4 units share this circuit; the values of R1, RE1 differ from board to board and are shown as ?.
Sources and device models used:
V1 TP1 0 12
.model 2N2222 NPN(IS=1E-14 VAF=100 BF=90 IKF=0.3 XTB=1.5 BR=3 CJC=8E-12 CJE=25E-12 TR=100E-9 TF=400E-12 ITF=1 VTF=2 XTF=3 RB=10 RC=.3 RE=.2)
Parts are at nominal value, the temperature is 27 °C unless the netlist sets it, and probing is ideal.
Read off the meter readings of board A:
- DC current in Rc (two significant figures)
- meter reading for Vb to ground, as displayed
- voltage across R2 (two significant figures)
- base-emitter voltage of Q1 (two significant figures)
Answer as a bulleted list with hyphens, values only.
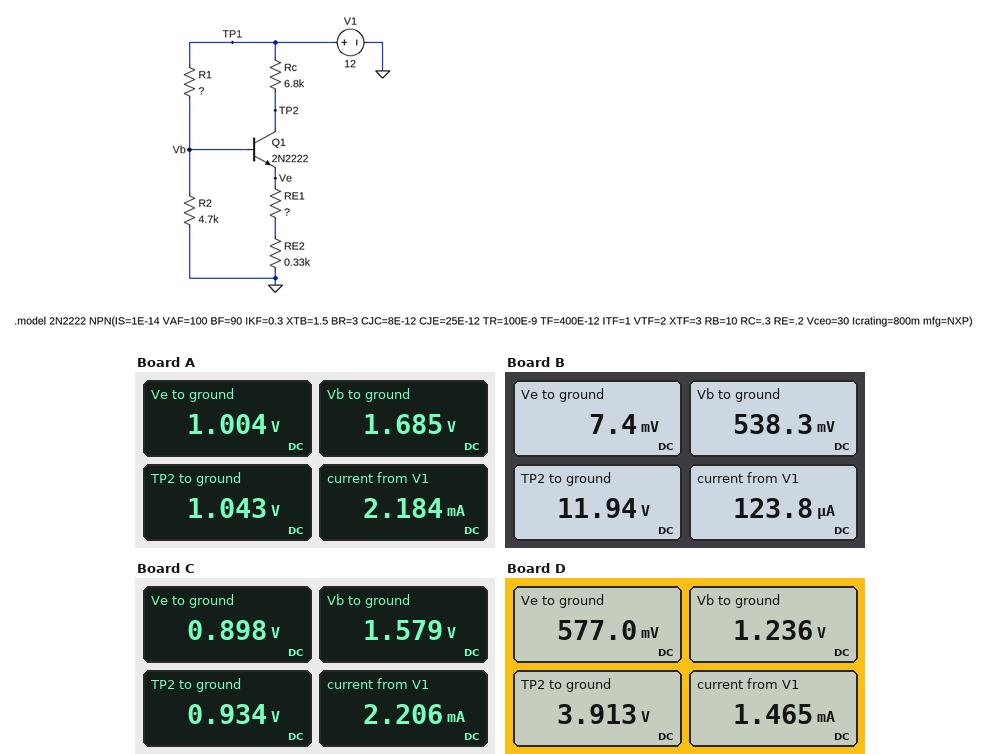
- 1.6 mA
- 1.685 V
- 1.7 V
- 680 mV
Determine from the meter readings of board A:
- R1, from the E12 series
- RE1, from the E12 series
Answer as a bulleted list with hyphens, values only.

- 18 kΩ
- 220 Ω
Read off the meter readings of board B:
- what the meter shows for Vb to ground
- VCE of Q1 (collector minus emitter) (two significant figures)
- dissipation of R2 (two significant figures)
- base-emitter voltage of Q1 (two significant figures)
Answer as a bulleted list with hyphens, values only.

- 538.3 mV
- 12 V
- 62 µW
- 530 mV
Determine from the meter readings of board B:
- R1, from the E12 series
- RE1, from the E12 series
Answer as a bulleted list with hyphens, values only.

- 100 kΩ
- 470 Ω
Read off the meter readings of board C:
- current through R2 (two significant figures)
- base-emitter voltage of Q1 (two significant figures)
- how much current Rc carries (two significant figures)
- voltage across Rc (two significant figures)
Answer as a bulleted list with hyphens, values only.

- 340 µA
- 680 mV
- 1.6 mA
- 11 V
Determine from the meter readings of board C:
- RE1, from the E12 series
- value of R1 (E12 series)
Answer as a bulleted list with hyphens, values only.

- 150 Ω
- 18 kΩ
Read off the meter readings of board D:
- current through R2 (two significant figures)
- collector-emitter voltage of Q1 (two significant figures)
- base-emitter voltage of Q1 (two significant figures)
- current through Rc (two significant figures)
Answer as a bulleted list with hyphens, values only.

- 260 µA
- 3.3 V
- 660 mV
- 1.2 mA
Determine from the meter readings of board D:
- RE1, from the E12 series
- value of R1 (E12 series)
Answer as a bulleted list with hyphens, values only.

- 150 Ω
- 39 kΩ
